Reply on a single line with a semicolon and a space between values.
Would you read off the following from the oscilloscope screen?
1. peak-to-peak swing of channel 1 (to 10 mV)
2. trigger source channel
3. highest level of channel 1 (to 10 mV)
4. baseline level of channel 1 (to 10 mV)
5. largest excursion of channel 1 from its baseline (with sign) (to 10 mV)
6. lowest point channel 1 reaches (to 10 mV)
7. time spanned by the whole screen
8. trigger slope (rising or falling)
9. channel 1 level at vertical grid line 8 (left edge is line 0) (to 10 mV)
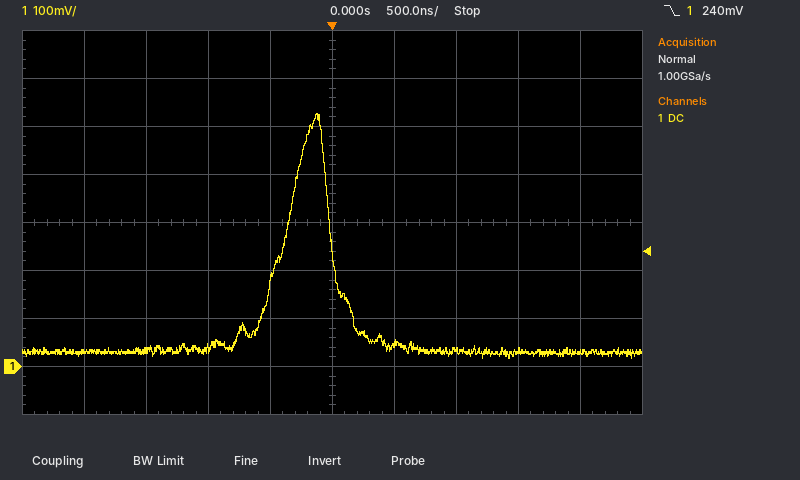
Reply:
510 mV; channel 1; 530 mV; 30 mV; +500 mV; 20 mV; 5 µs; falling; 30 mV
